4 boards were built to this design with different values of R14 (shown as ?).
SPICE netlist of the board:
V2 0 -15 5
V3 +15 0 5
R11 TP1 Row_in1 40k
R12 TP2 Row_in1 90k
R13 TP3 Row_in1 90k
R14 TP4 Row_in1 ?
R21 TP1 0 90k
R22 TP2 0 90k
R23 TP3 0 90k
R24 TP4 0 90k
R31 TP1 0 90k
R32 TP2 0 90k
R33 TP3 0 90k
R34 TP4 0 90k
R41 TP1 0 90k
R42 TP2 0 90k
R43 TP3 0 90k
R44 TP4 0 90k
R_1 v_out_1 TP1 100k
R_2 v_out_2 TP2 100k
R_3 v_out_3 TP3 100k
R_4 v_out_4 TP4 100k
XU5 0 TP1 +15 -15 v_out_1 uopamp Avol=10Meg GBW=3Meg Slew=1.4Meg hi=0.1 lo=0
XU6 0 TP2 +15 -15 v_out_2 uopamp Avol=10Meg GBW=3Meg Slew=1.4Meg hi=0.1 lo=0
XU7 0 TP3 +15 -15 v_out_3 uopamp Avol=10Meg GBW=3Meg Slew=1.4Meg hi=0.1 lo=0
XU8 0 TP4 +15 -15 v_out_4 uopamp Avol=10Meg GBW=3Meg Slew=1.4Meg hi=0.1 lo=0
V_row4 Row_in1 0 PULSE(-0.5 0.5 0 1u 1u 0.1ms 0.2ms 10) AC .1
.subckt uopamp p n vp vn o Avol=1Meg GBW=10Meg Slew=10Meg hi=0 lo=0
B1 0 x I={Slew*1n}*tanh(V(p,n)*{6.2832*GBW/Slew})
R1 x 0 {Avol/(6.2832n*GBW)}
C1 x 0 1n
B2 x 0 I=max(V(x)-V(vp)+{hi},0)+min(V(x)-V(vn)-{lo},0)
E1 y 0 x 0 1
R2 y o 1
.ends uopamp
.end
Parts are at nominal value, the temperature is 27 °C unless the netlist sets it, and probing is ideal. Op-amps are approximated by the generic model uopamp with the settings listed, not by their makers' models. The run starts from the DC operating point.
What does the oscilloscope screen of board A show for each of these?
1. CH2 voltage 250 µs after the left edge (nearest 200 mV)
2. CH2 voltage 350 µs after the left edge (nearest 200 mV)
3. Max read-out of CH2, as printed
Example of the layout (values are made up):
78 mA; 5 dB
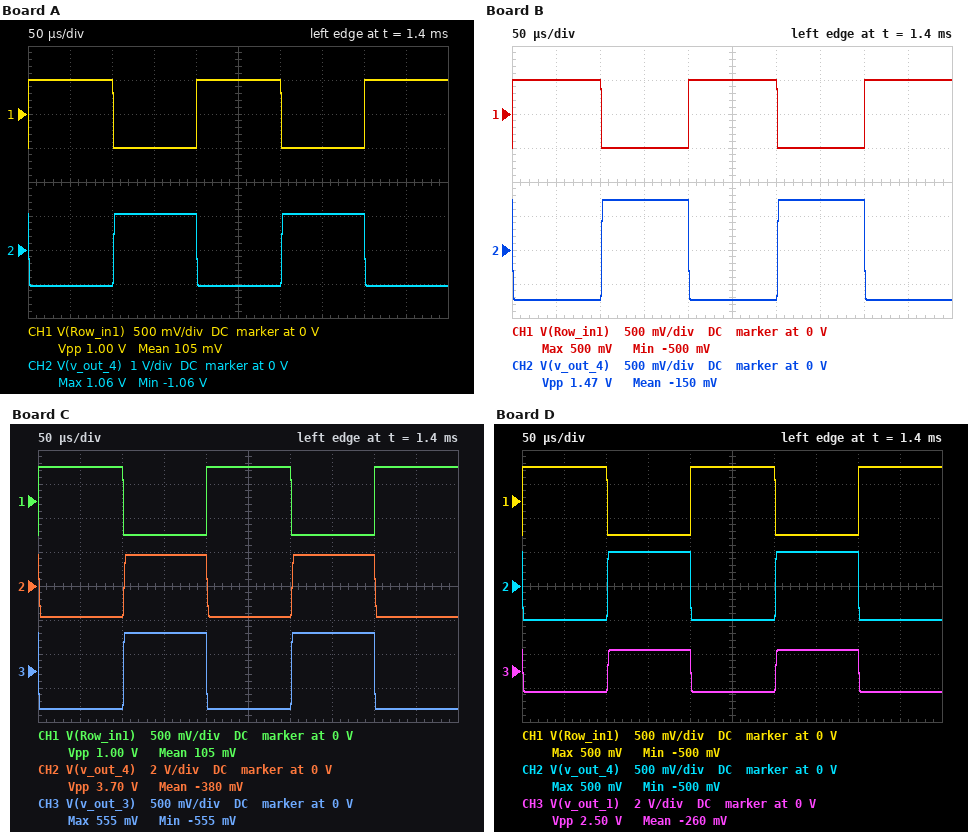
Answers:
-1.0 V; 1.0 V; 1.06 V
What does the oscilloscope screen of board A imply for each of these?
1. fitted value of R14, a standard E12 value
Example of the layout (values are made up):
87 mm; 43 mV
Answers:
47 kΩ
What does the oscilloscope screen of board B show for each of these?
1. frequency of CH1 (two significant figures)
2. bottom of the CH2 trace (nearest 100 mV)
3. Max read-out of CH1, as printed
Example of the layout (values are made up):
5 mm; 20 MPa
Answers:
5.0 kHz; -700 mV; 500 mV
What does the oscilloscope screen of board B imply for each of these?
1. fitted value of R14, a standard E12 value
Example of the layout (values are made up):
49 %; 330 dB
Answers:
68 kΩ
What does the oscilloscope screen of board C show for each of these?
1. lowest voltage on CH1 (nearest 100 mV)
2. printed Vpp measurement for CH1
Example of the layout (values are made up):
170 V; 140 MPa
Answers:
-500 mV; 1.00 V
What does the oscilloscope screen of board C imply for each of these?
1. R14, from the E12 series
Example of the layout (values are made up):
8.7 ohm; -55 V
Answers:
27 kΩ
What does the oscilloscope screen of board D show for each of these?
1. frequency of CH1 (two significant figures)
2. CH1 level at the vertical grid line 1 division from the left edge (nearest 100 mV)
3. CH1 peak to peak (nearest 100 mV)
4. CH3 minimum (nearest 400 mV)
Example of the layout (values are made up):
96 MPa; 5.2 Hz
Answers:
5.0 kHz; 500 mV; 1.0 V; -1.2 V
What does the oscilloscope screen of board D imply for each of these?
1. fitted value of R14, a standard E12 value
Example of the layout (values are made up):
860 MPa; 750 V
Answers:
100 kΩ
